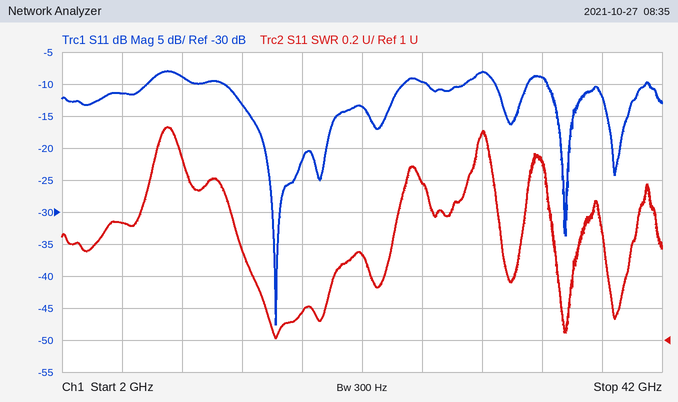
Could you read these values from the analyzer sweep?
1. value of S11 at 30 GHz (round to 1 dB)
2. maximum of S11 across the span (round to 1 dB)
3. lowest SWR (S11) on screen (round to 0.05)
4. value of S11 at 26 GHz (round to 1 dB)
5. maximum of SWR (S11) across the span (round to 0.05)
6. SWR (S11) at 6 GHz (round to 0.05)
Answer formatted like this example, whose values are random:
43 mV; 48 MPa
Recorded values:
-8 dB; -8 dB; 1.00; -10 dB; 2.35; 1.75
